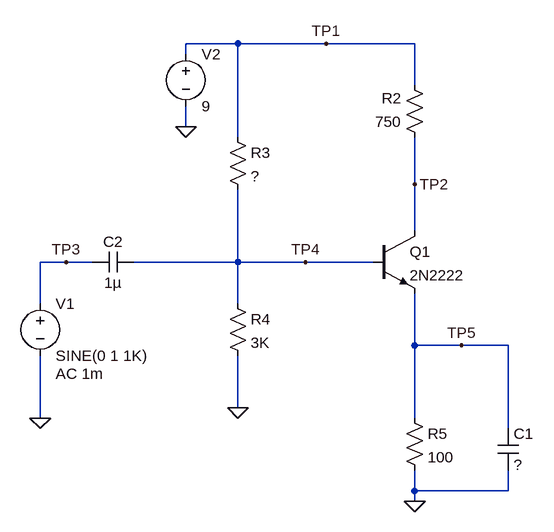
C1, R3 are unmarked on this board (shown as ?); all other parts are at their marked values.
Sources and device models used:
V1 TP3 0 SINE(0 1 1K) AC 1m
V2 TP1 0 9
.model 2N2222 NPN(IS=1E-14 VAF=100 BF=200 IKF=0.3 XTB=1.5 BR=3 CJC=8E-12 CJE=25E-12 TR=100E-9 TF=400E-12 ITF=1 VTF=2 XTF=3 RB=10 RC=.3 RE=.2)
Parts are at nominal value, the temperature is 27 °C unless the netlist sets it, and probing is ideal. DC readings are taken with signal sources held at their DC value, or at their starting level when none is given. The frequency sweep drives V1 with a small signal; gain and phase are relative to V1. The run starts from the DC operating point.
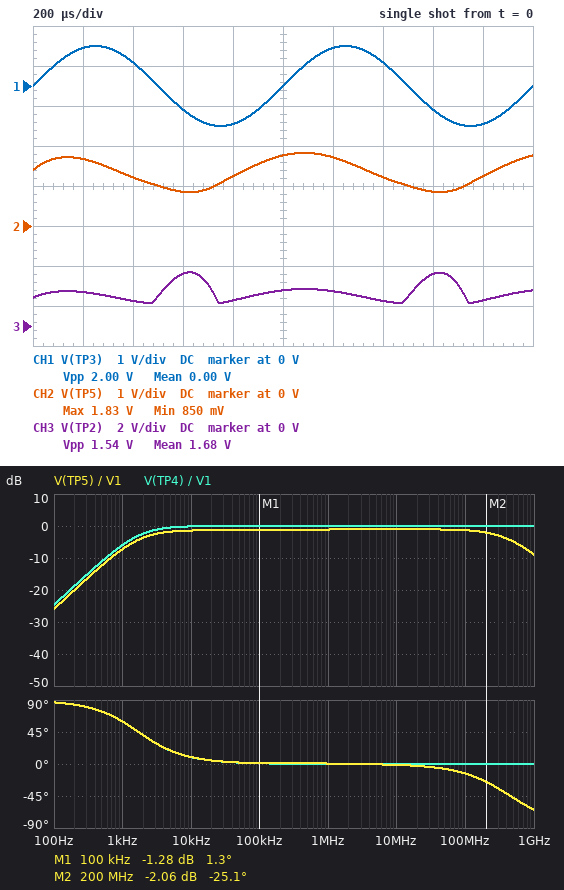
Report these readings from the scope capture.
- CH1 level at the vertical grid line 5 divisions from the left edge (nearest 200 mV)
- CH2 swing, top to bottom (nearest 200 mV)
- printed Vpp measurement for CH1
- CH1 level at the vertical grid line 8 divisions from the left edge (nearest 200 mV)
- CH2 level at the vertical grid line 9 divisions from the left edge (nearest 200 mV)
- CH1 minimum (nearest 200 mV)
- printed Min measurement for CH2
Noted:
0 V
1.0 V
2.00 V
-600 mV
1.2 V
-1.0 V
850 mV
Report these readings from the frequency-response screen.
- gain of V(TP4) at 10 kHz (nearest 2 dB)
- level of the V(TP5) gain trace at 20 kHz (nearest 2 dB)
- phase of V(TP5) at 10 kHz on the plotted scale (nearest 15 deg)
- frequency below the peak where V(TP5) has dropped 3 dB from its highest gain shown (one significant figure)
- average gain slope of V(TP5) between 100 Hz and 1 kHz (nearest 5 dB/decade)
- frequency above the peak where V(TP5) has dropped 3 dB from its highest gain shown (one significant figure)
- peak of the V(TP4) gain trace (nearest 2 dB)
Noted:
0 dB
-2 dB
15 deg
2 kHz
20 dB/decade
400 MHz
0 dB
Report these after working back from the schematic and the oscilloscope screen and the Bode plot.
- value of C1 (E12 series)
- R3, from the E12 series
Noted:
39 pF
1.5 kΩ
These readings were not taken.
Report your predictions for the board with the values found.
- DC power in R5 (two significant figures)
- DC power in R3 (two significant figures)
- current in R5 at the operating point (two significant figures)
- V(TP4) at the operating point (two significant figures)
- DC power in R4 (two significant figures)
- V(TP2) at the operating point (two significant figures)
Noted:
19 mW
31 mW
14 mA
2.2 V
1.6 mW
1.4 V
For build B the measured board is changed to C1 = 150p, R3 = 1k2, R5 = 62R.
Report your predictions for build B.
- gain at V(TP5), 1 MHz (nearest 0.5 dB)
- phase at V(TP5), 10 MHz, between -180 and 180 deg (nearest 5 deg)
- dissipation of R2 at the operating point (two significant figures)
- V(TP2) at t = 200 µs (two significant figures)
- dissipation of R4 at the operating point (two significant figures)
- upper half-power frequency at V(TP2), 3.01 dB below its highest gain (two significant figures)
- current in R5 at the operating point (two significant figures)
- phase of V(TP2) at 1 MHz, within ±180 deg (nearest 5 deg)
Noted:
-1.5 dB
-5 deg
85 mW
1.2 V
1.1 mW
120 MHz
16 mA
0 deg
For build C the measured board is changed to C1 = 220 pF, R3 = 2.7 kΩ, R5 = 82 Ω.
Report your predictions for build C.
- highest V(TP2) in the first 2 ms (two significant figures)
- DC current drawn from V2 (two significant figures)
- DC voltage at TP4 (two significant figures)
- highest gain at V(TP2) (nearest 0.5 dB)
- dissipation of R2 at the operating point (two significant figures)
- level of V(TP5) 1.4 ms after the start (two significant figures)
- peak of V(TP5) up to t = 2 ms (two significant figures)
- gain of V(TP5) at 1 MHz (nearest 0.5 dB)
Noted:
7.8 V
13 mA
1.8 V
-1.0 dB
84 mW
860 mV
1.4 V
-1.5 dB
